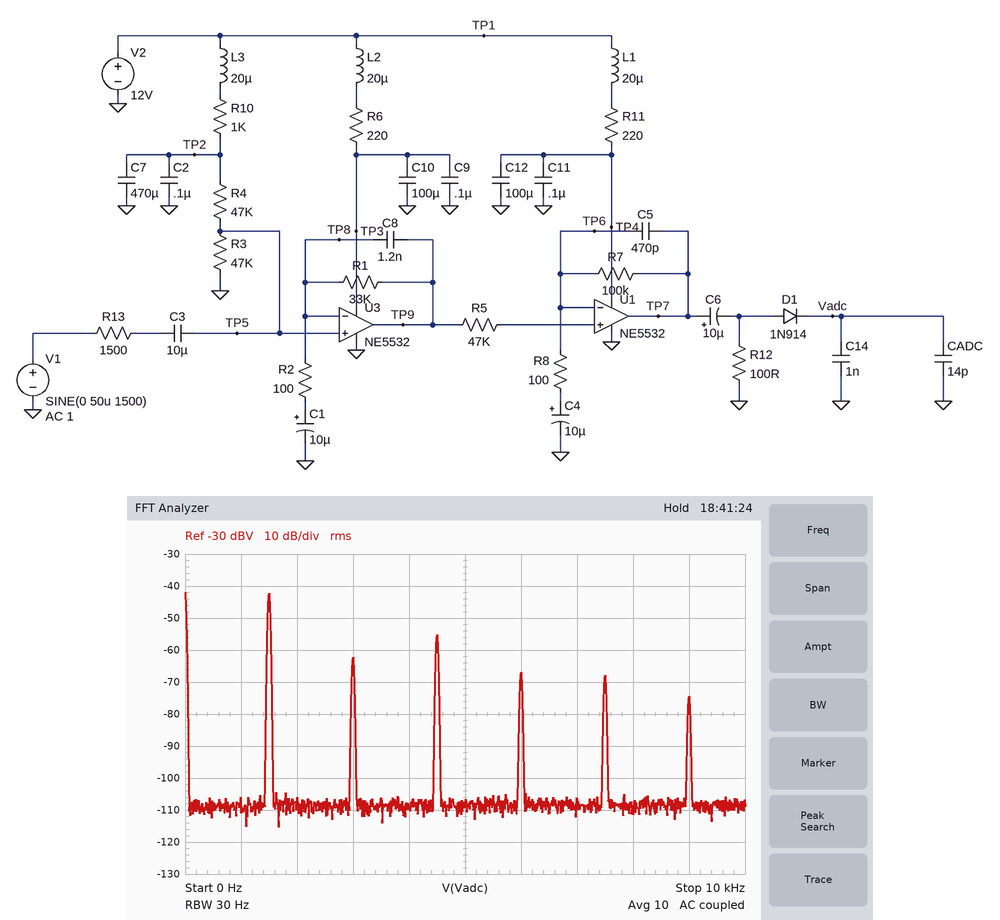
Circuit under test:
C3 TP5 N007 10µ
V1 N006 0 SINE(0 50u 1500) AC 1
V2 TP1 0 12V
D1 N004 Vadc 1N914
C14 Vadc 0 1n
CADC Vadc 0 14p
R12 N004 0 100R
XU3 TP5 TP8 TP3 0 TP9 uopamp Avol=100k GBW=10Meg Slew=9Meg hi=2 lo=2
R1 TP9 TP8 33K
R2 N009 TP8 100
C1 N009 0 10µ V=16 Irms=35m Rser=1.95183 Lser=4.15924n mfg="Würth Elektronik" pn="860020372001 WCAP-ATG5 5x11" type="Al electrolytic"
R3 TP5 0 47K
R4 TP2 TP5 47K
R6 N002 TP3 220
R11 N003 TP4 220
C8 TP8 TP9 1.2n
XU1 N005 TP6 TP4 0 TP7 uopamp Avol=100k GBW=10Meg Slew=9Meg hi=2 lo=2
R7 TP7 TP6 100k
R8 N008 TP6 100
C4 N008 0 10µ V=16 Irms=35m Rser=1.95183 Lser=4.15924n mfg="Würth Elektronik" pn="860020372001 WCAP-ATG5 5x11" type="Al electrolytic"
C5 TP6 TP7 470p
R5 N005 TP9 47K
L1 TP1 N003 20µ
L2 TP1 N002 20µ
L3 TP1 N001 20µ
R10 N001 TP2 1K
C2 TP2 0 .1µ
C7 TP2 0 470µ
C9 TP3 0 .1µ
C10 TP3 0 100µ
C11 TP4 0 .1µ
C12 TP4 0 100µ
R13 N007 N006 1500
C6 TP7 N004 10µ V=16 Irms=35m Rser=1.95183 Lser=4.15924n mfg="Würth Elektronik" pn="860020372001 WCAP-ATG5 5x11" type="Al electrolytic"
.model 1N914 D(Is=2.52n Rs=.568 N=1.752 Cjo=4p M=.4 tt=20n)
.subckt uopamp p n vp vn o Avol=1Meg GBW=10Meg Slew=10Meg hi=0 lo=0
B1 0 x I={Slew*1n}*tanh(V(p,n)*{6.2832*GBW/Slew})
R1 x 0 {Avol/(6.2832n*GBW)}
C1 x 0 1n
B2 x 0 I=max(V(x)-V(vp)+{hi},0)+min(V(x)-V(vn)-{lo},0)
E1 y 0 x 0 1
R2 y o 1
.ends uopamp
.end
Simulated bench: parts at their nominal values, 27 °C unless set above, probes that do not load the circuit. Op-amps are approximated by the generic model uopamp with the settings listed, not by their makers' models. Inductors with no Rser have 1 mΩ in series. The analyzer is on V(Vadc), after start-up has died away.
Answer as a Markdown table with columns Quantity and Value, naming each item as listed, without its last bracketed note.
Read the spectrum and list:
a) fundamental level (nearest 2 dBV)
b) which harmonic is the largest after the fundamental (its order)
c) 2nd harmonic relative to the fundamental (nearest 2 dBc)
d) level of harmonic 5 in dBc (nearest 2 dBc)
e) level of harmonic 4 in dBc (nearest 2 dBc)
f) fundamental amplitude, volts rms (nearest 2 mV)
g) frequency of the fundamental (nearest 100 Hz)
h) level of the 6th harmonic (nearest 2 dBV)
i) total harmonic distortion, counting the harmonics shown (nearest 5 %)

| Quantity | Value |
|---|---|
| fundamental level | -42 dBV |
| which harmonic is the largest after the fundamental | 3 |
| 2nd harmonic relative to the fundamental | -20 dBc |
| level of harmonic 5 in dBc | -26 dBc |
| level of harmonic 4 in dBc | -24 dBc |
| fundamental amplitude, volts rms | 8 mV |
| frequency of the fundamental | 1.5 kHz |
| level of the 6th harmonic | -74 dBV |
| total harmonic distortion, counting the harmonics shown | 25 % |
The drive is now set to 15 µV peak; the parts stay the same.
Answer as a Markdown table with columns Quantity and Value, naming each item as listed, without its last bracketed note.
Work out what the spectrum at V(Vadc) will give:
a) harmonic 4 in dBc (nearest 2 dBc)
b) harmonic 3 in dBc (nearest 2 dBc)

| Quantity | Value |
|---|---|
| harmonic 4 in dBc | -36 dBc |
| harmonic 3 in dBc | -30 dBc |
